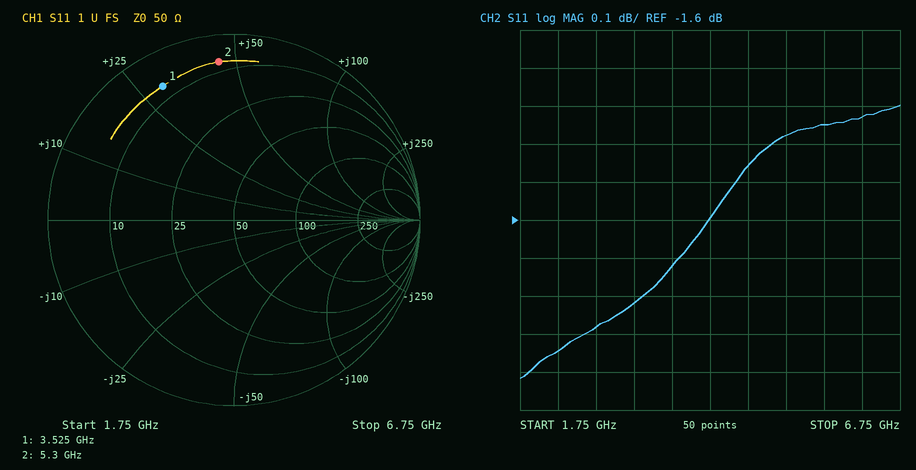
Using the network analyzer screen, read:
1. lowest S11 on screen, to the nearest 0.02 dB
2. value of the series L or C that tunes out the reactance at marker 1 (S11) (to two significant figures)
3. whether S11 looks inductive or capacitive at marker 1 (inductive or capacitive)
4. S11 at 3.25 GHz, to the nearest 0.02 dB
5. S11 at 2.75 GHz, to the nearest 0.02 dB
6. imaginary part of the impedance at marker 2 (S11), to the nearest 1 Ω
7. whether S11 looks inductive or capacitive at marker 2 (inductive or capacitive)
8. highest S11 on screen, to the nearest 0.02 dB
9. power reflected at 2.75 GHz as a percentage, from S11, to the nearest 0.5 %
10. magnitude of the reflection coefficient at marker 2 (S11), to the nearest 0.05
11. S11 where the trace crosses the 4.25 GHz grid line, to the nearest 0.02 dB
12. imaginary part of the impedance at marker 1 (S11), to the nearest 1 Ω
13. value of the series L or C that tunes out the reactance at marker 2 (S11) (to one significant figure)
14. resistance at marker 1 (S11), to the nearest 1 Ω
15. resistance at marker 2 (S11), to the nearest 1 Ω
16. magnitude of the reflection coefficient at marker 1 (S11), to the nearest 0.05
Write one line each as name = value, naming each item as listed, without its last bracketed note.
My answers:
lowest S11 on screen, to the nearest 0.02 dB = -2.02 dB
value of the series L or C that tunes out the reactance at marker 1 (S11) = 1.5 pF
whether S11 looks inductive or capacitive at marker 1 = inductive
S11 at 3.25 GHz, to the nearest 0.02 dB = -1.82 dB
S11 at 2.75 GHz, to the nearest 0.02 dB = -1.88 dB
imaginary part of the impedance at marker 2 (S11), to the nearest 1 Ω = +45 Ω
whether S11 looks inductive or capacitive at marker 2 = inductive
highest S11 on screen, to the nearest 0.02 dB = -1.30 dB
power reflected at 2.75 GHz as a percentage, from S11, to the nearest 0.5 % = 65.0 %
magnitude of the reflection coefficient at marker 2 (S11), to the nearest 0.05 = 0.85
S11 where the trace crosses the 4.25 GHz grid line, to the nearest 0.02 dB = -1.60 dB
imaginary part of the impedance at marker 1 (S11), to the nearest 1 Ω = +30 Ω
value of the series L or C that tunes out the reactance at marker 2 (S11) = 700 fF
resistance at marker 1 (S11), to the nearest 1 Ω = 7 Ω
resistance at marker 2 (S11), to the nearest 1 Ω = 7 Ω
magnitude of the reflection coefficient at marker 1 (S11), to the nearest 0.05 = 0.80
